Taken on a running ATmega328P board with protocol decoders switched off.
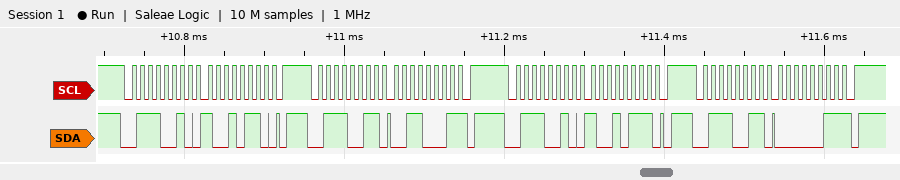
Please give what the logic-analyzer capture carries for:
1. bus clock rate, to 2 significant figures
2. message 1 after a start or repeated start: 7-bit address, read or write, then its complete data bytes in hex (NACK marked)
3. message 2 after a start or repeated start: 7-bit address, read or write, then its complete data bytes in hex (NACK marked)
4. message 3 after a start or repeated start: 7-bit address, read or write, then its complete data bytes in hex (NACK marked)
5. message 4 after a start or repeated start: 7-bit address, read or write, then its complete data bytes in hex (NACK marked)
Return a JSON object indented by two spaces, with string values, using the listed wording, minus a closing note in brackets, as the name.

{
  "bus clock rate, to 2 significant figures": "100 kHz",
  "message 1 after a start or repeated start: 7-bit address, read or write, then its complete data bytes in hex": "0x39 write: 96",
  "message 2 after a start or repeated start: 7-bit address, read or write, then its complete data bytes in hex": "0x39 read: 31 NACK",
  "message 3 after a start or repeated start: 7-bit address, read or write, then its complete data bytes in hex": "0x39 write: 97",
  "message 4 after a start or repeated start: 7-bit address, read or write, then its complete data bytes in hex": "0x39 read: 03 NACK"
}
